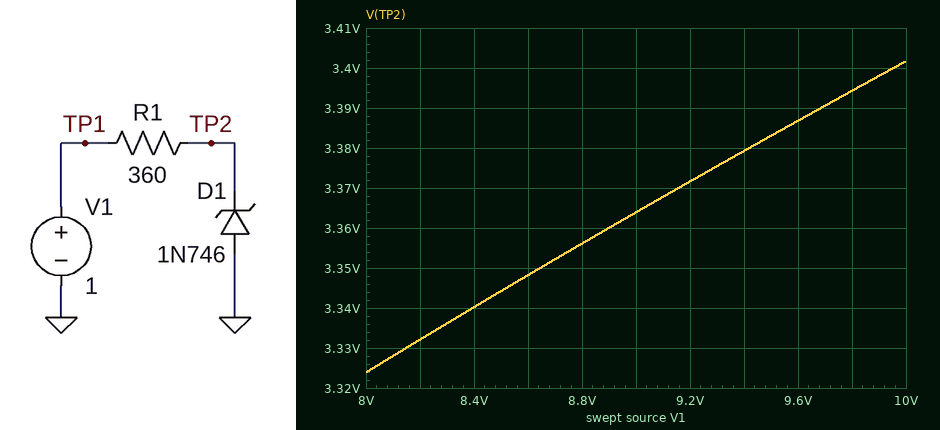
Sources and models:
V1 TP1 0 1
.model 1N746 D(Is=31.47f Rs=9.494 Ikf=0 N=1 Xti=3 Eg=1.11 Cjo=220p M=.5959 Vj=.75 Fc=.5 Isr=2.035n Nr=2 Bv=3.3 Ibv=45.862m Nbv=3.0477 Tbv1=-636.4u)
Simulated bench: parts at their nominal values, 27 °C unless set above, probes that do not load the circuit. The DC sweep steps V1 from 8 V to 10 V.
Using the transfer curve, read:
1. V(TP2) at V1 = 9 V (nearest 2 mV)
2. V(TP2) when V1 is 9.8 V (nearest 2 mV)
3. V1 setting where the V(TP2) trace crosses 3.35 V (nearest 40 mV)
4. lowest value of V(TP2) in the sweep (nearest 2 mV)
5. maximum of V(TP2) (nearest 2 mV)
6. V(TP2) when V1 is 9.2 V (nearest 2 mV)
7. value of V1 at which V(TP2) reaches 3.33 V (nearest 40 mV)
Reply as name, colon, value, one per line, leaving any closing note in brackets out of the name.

V(TP2) at V1 = 9 V: 3.364 V
V(TP2) when V1 is 9.8 V: 3.394 V
V1 setting where the V(TP2) trace crosses 3.35 V: 8.64 V
lowest value of V(TP2) in the sweep: 3.324 V
maximum of V(TP2): 3.402 V
V(TP2) when V1 is 9.2 V: 3.372 V
value of V1 at which V(TP2) reaches 3.33 V: 8.16 V
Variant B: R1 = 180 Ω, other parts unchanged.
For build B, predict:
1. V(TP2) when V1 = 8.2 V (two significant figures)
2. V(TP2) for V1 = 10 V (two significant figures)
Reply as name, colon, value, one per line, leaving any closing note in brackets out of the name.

V(TP2) when V1 = 8.2 V: 3.5 V
V(TP2) for V1 = 10 V: 3.6 V
